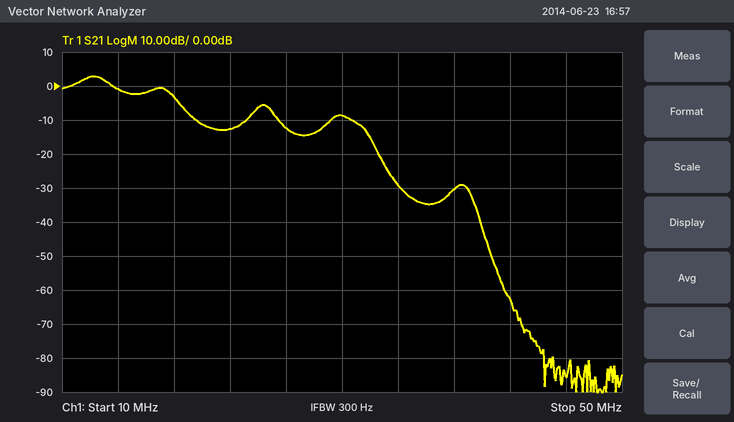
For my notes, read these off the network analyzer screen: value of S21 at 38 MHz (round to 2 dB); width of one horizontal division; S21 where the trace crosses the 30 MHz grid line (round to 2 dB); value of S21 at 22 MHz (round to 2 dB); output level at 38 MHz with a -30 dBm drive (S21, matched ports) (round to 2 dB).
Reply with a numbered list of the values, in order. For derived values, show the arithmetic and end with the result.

1. -30 dB
2. 4 MHz
3. -8 dB
4. -12 dB
5. -30 dBm + (-30 dB) = -60 dBm
